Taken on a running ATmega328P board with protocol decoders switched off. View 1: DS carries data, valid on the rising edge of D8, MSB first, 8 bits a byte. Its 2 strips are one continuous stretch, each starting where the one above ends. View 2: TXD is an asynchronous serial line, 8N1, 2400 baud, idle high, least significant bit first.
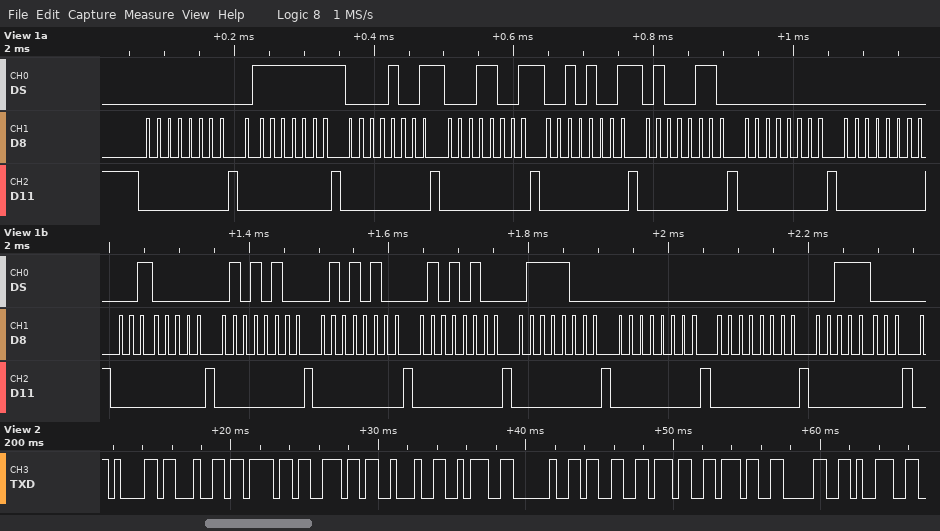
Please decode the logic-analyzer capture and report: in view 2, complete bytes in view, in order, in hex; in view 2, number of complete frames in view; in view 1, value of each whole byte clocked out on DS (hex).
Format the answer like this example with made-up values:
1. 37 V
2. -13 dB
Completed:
1. 61 64 6F 6E 22 3A 20 33 37 37 30 39
2. 12
3. 00 7F 09 19 29 46 00 00 20 54 54 54 78 00 00 38
